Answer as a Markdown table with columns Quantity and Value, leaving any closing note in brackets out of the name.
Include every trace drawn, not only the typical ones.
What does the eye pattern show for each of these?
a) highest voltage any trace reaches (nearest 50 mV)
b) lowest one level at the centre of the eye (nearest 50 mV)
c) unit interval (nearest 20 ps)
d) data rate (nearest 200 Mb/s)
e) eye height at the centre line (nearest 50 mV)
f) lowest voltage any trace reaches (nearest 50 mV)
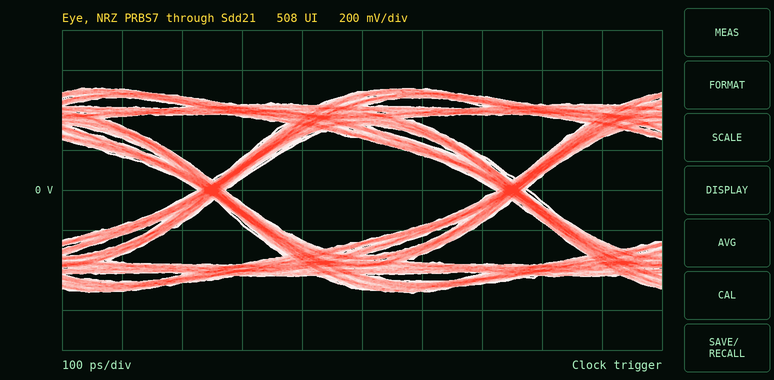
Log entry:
| Quantity | Value |
|---|---|
| highest voltage any trace reaches | 500 mV |
| lowest one level at the centre of the eye | 250 mV |
| unit interval | 500 ps |
| data rate | 2.0 Gb/s |
| eye height at the centre line | 500 mV |
| lowest voltage any trace reaches | -500 mV |
